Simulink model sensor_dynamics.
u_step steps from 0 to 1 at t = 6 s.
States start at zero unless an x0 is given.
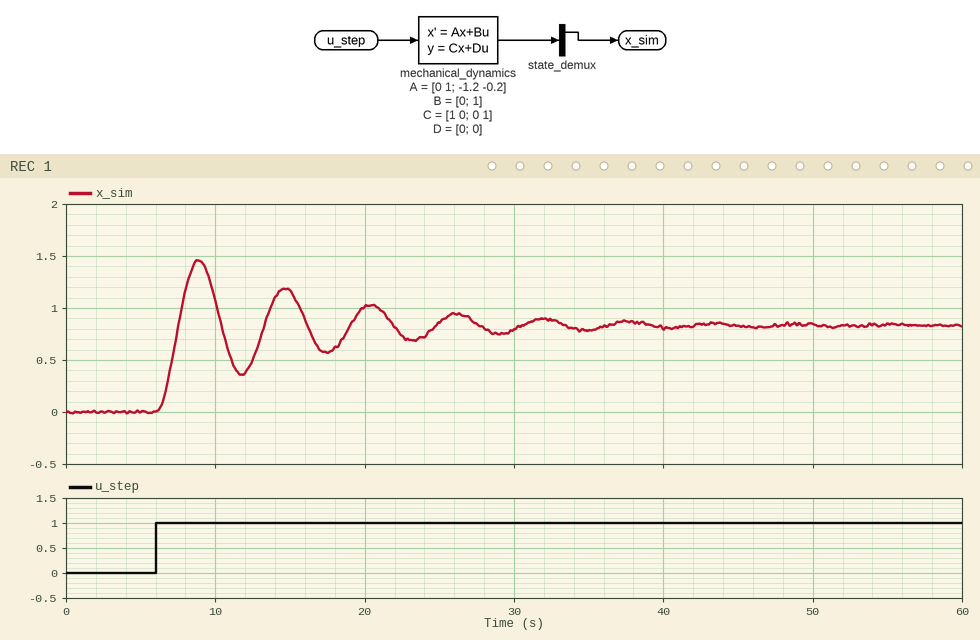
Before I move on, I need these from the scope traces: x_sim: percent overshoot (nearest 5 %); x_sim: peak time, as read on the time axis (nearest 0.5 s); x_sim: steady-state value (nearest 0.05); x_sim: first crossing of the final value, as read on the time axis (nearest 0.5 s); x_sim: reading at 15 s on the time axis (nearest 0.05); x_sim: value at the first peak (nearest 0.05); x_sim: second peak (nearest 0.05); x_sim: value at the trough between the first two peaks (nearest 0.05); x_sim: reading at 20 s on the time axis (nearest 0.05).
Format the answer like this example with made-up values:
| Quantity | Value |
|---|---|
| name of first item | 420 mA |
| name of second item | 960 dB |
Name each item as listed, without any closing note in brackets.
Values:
| Quantity | Value |
|---|---|
| x_sim: percent overshoot | 75 % |
| x_sim: peak time, as read on the time axis | 9.0 s |
| x_sim: steady-state value | 0.85 |
| x_sim: first crossing of the final value, as read on the time axis | 7.5 s |
| x_sim: reading at 15 s on the time axis | 1.15 |
| x_sim: value at the first peak | 1.45 |
| x_sim: second peak | 1.20 |
| x_sim: value at the trough between the first two peaks | 0.35 |
| x_sim: reading at 20 s on the time axis | 1.00 |
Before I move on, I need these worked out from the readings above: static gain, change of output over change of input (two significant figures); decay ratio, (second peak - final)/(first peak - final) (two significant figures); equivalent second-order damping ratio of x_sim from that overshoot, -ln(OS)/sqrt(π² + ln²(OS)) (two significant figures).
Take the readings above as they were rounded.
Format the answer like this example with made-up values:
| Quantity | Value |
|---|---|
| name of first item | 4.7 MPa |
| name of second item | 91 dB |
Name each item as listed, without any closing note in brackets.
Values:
| Quantity | Value |
|---|---|
| static gain, change of output over change of input | 0.85 |
| decay ratio, (second peak - final)/(first peak - final) | 0.58 |
| equivalent second-order damping ratio of x_sim from that overshoot, -ln(OS)/sqrt(π² + ln²(OS)) | 0.091 |
